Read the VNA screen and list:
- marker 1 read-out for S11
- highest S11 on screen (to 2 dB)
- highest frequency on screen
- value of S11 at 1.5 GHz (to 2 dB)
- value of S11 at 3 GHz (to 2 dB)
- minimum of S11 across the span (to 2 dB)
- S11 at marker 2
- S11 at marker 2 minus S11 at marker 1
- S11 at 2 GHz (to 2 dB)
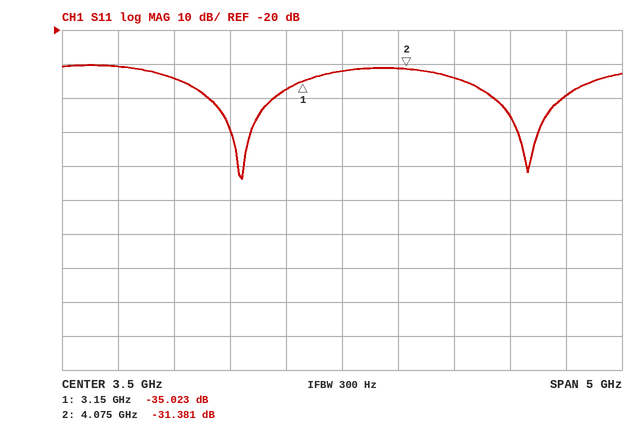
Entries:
-35.023 dB
-30 dB
6 GHz
-30 dB
-38 dB
-64 dB
-31.381 dB
3.642 dB
-34 dB
